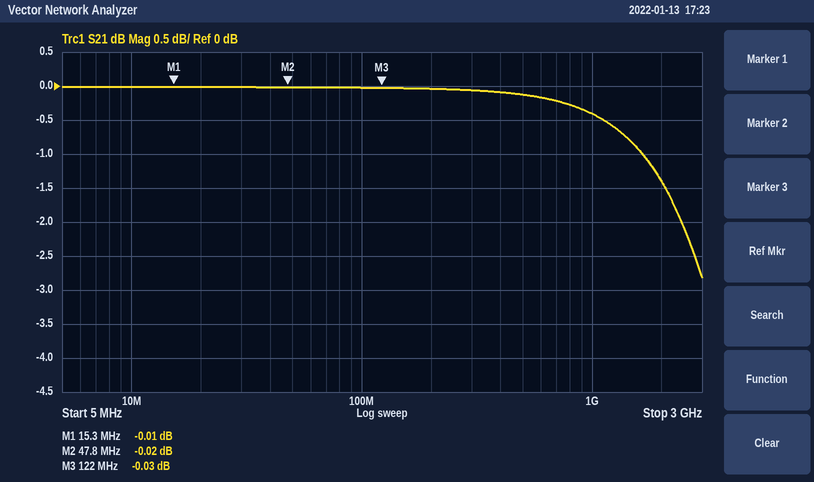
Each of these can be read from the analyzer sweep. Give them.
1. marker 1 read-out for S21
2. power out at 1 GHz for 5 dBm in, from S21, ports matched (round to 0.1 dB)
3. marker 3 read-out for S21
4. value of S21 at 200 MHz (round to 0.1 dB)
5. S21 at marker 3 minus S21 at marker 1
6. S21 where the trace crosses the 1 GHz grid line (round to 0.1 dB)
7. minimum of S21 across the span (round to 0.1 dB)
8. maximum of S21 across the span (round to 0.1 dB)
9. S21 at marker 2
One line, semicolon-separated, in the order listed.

-0.01 dB; 4.6 dBm; -0.03 dB; 0.0 dB; -0.02 dB; -0.4 dB; -2.8 dB; 0.0 dB; -0.02 dB
